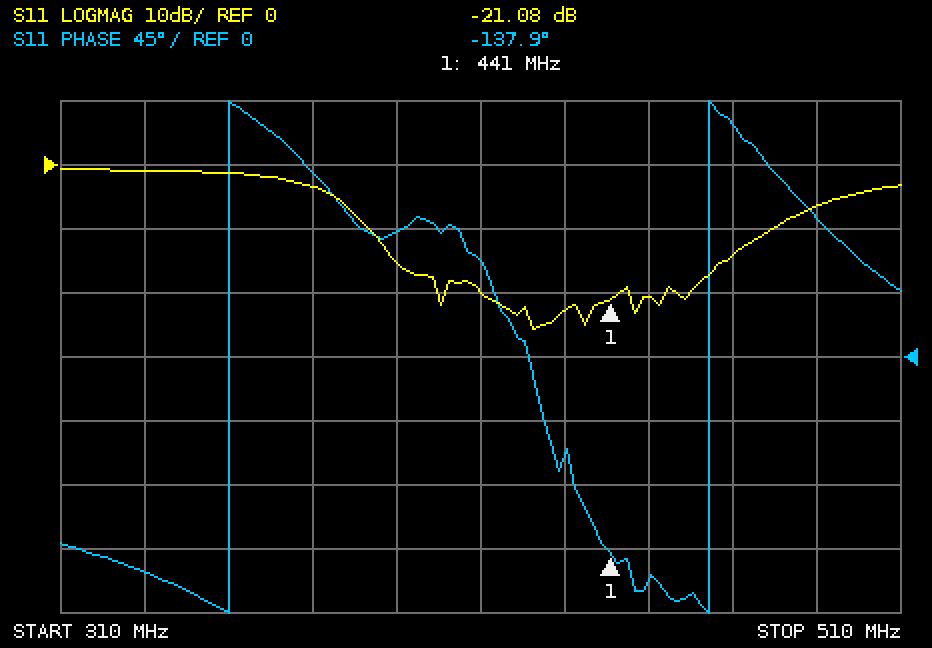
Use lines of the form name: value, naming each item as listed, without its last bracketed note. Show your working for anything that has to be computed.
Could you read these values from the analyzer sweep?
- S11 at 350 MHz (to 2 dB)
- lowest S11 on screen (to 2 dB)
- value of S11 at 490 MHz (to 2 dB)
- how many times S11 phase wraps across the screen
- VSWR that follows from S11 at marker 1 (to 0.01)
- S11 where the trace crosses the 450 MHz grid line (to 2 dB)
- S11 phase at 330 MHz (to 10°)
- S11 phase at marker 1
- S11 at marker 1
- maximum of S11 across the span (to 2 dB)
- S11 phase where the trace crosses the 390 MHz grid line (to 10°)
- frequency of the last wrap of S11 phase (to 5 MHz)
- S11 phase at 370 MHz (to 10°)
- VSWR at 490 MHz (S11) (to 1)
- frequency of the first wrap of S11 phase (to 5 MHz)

S11 at 350 MHz: -2 dB
lowest S11 on screen: -26 dB
value of S11 at 490 MHz: -6 dB
how many times S11 phase wraps across the screen: 2
VSWR that follows from S11 at marker 1: (1 + 0.0883)/(1 − 0.0883) ≈ 1.19
S11 where the trace crosses the 450 MHz grid line: -20 dB
S11 phase at 330 MHz: -150°
S11 phase at marker 1: -137.9°
S11 at marker 1: -21.08 dB
maximum of S11 across the span: 0 dB
S11 phase where the trace crosses the 390 MHz grid line: 90°
frequency of the last wrap of S11 phase: 465 MHz
S11 phase at 370 MHz: 130°
VSWR at 490 MHz (S11): |Γ| = 10^(-6/20) = 0.5012; VSWR = (1 + 0.5012)/(1 − 0.5012) ≈ 3
frequency of the first wrap of S11 phase: 350 MHz
